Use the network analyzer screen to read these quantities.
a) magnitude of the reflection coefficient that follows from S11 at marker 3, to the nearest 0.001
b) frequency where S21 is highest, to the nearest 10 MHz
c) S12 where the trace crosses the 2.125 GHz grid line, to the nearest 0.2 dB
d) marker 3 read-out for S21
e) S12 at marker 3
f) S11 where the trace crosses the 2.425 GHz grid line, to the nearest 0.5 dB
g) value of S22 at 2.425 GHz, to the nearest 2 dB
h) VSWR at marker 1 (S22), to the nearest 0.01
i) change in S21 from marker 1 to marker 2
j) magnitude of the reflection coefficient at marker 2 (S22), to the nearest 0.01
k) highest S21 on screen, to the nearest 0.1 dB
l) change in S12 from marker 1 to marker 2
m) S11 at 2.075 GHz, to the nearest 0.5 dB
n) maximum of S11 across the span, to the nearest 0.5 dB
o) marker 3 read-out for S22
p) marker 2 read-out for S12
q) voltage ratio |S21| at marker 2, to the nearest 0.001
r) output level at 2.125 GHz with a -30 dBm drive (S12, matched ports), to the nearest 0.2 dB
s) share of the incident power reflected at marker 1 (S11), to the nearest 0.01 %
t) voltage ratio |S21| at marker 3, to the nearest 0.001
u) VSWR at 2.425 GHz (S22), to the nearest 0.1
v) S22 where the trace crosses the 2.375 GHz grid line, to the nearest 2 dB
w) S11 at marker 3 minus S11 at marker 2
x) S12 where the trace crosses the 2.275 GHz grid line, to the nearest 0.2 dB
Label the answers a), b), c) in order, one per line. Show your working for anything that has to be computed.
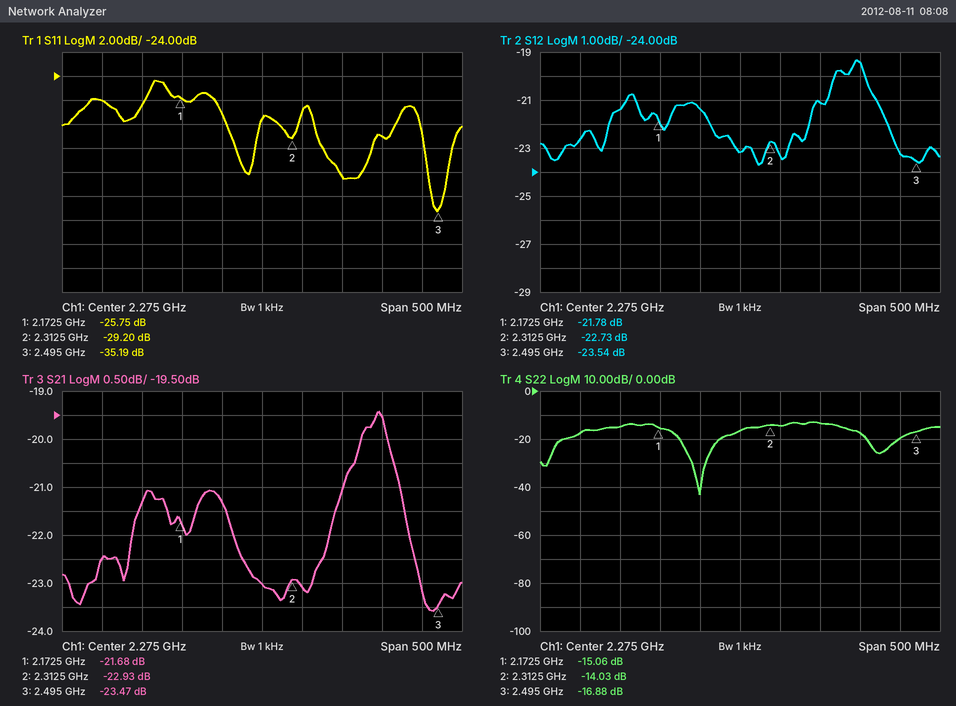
a) 10^(-35.19/20) ≈ 0.017
b) 2.42 GHz
c) -21.4 dB
d) -23.47 dB
e) -23.54 dB
f) -29.0 dB
g) -18 dB
h) (1 + 0.1766)/(1 − 0.1766) ≈ 1.43
i) -22.93 − (-21.68) = -1.25 dB
j) 10^(-14.03/20) ≈ 0.20
k) -19.4 dB
l) -22.73 − (-21.78) = -0.95 dB
m) -26.0 dB
n) -24.5 dB
o) -16.88 dB
p) -22.73 dB
q) 10^(-22.93/20) ≈ 0.071
r) -30 dBm + (-21.4 dB) = -51.4 dBm
s) 10^(-25.75/10) ≈ 0.27 %
t) 10^(-23.47/20) ≈ 0.067
u) |Γ| = 10^(-18/20) = 0.1259; VSWR = (1 + 0.1259)/(1 − 0.1259) ≈ 1.3
v) -14 dB
w) -35.19 − (-29.2) = -5.99 dB
x) -23.2 dB
